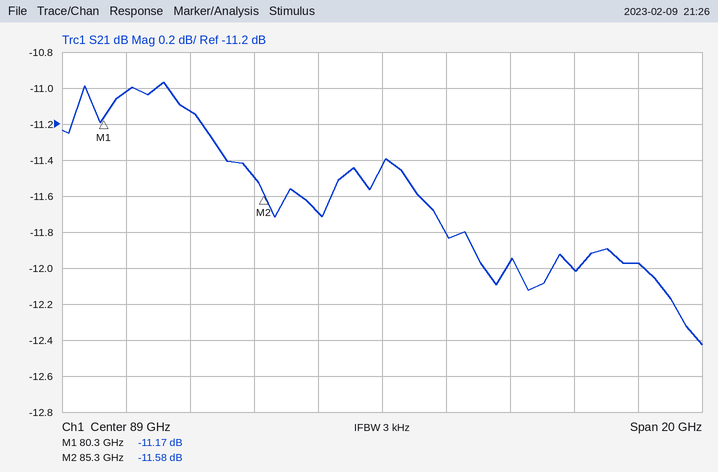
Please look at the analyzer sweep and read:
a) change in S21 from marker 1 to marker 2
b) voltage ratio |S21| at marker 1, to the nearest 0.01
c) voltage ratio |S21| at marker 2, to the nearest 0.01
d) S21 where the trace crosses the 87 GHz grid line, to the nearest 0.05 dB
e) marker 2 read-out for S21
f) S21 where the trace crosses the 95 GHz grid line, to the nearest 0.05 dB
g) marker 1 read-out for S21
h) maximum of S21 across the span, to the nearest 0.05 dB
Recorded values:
-0.41 dB
0.28
0.26
-11.70 dB
-11.58 dB
-12.00 dB
-11.17 dB
-10.95 dB
